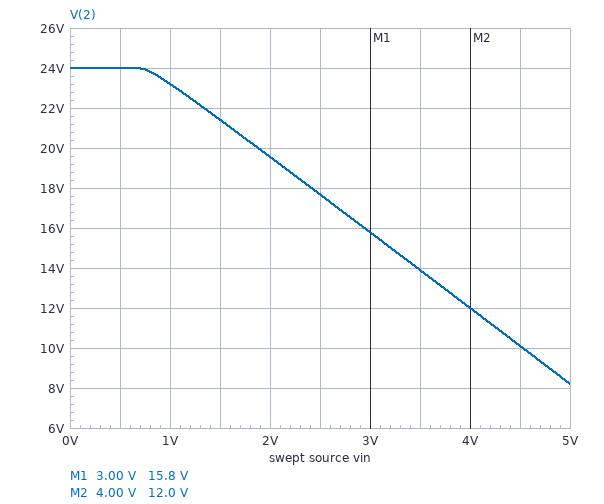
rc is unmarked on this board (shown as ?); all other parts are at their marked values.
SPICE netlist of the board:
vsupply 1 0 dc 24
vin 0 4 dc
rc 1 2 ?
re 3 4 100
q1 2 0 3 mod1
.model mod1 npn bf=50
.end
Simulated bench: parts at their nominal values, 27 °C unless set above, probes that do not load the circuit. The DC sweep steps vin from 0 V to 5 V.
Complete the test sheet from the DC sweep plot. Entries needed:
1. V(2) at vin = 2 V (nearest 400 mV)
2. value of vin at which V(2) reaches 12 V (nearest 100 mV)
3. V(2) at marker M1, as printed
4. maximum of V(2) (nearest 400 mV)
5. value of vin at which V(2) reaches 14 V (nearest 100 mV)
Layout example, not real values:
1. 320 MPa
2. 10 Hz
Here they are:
1. 19.6 V
2. 4.0 V
3. 15.8 V
4. 24.0 V
5. 3.5 V
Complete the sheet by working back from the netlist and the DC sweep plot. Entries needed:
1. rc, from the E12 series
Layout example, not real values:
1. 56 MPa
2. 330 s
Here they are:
1. 390 Ω
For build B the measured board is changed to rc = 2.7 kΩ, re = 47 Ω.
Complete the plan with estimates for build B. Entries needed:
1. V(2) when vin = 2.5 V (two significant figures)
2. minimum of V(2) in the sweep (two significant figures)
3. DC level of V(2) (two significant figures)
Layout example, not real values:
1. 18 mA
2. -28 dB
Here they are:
1. -860 mV
2. -890 mV
3. 24 V
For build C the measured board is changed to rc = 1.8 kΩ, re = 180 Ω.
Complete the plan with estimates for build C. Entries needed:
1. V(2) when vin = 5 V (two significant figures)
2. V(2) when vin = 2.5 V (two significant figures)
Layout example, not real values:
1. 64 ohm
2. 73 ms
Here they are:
1. -830 mV
2. 7.6 V
